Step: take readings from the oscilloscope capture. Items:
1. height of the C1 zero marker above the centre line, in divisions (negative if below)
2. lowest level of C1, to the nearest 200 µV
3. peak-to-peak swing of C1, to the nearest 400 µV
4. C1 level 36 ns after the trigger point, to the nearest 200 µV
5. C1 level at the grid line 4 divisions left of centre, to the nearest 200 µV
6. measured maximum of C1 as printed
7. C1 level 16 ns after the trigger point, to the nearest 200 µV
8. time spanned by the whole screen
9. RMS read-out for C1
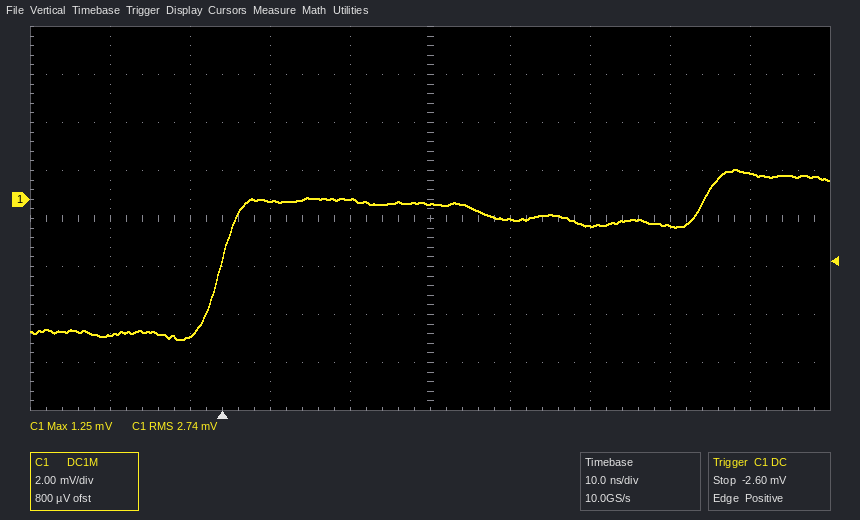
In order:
+0.4 div
-5.8 mV
7.2 mV
-800 µV
-5.6 mV
1.25 mV
0.0 mV
100 ns
2.74 mV
